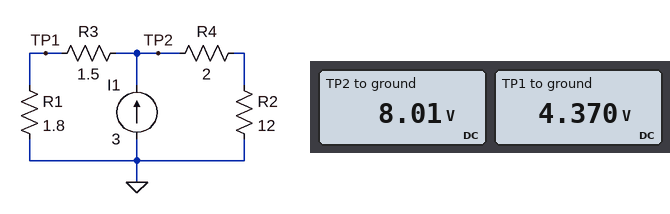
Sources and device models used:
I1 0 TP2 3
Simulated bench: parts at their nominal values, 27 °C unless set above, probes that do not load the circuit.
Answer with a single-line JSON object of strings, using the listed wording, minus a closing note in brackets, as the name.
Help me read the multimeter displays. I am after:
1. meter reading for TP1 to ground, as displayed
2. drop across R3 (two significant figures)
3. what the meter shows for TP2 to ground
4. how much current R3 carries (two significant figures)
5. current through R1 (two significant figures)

{"meter reading for TP1 to ground, as displayed": "4.370 V", "drop across R3": "3.6 V", "what the meter shows for TP2 to ground": "8.01 V", "how much current R3 carries": "2.4 A", "current through R1": "2.4 A"}
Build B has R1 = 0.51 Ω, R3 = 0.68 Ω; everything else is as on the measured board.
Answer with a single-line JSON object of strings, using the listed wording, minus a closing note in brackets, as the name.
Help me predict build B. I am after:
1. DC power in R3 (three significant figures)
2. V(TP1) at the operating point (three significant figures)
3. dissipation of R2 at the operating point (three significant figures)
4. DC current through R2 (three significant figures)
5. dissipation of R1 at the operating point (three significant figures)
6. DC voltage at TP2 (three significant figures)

{"DC power in R3": "5.20 W", "V(TP1) at the operating point": "1.41 V", "dissipation of R2 at the operating point": "663 mW", "DC current through R2": "235 mA", "dissipation of R1 at the operating point": "3.90 W", "DC voltage at TP2": "3.29 V"}
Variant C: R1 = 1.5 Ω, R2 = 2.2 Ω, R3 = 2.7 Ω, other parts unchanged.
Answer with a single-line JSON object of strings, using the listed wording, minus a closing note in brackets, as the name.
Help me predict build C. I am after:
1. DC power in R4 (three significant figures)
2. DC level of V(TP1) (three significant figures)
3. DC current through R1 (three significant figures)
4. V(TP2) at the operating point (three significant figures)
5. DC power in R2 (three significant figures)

{"DC power in R4": "4.50 W", "DC level of V(TP1)": "2.25 V", "DC current through R1": "1.50 A", "V(TP2) at the operating point": "6.30 V", "DC power in R2": "4.95 W"}
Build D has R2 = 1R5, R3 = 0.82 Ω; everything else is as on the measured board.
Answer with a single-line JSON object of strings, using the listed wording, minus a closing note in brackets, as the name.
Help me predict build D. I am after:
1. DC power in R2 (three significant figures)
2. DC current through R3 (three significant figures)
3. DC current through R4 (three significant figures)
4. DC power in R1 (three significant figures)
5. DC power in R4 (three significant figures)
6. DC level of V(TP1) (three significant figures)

{"DC power in R2": "2.47 W", "DC current through R3": "1.72 A", "DC current through R4": "1.28 A", "DC power in R1": "5.30 W", "DC power in R4": "3.30 W", "DC level of V(TP1)": "3.09 V"}
